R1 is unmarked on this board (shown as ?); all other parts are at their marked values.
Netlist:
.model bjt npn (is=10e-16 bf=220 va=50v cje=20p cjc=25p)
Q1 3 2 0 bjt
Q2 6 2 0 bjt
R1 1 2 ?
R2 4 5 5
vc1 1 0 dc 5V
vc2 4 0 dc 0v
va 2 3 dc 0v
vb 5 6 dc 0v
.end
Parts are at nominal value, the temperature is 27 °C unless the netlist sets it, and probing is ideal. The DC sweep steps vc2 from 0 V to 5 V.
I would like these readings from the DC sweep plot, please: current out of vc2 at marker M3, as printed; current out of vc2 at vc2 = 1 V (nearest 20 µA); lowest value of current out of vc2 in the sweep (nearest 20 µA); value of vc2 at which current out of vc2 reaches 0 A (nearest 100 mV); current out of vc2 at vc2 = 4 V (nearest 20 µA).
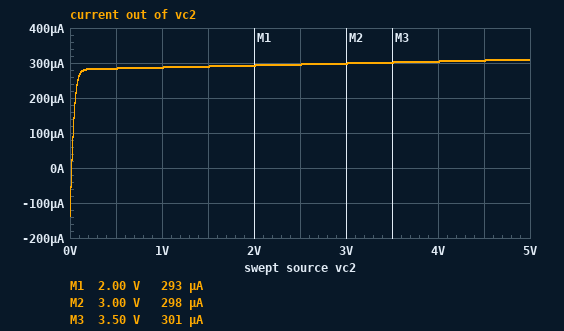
301 µA
280 µA
-140 µA
0 V
300 µA
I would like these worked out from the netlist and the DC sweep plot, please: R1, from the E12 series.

15 kΩ
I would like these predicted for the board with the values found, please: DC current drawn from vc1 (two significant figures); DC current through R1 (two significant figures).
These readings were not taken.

290 µA
290 µA
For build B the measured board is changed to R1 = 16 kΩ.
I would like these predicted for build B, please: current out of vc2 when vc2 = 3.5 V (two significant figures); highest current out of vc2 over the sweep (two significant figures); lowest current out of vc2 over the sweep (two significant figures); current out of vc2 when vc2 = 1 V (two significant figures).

280 µA
290 µA
-130 µA
270 µA
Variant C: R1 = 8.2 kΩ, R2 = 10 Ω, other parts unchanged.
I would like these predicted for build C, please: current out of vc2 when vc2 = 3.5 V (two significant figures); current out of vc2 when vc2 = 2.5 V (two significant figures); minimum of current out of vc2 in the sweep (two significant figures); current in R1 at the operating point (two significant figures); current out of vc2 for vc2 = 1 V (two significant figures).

550 µA
540 µA
-230 µA
530 µA
520 µA
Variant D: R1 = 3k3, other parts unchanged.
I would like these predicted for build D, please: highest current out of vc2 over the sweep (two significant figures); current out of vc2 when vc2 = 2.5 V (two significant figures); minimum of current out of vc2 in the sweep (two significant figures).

1.4 mA
1.3 mA
-550 µA
